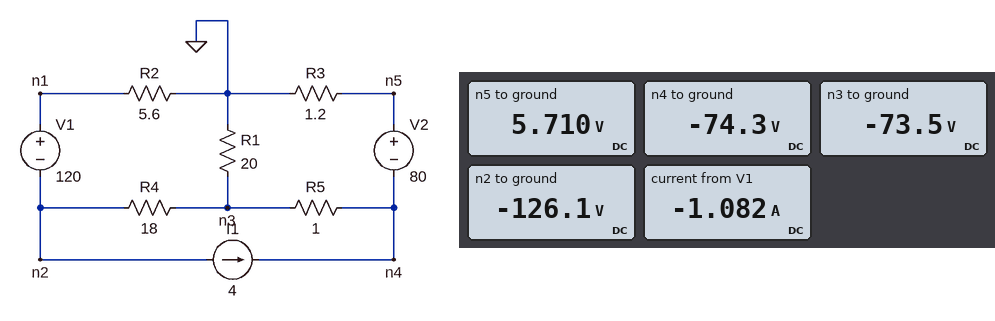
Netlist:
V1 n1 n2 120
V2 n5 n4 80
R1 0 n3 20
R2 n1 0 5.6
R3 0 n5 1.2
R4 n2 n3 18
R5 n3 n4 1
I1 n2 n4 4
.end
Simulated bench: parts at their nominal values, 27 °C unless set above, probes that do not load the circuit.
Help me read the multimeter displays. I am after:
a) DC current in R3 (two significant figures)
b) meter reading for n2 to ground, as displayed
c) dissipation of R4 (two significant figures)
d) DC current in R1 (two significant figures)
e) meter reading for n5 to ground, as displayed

4.8 A
-126.1 V
150 W
3.7 A
5.710 V
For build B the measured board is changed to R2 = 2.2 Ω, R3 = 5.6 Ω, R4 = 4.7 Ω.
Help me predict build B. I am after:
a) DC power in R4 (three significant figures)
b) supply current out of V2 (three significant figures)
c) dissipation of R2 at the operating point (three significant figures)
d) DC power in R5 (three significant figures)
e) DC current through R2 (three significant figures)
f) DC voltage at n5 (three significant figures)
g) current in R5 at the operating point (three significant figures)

244 W
747 mA
22.6 W
10.6 W
3.21 A
4.18 V
3.25 A
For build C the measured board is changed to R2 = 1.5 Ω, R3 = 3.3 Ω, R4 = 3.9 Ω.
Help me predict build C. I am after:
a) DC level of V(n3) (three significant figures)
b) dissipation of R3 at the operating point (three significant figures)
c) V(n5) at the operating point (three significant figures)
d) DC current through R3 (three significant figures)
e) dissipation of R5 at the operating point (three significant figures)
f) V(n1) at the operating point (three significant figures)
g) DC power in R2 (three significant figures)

-83.1 V
145 mW
693 mV
210 mA
14.4 W
5.92 V
23.3 W
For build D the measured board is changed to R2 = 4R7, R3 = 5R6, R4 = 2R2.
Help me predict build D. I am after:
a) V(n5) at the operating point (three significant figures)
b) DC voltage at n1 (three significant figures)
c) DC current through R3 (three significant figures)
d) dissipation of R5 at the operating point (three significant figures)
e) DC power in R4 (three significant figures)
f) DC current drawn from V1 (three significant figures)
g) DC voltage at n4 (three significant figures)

632 mV
19.0 V
113 mA
15.1 W
143 W
4.05 A
-79.4 V
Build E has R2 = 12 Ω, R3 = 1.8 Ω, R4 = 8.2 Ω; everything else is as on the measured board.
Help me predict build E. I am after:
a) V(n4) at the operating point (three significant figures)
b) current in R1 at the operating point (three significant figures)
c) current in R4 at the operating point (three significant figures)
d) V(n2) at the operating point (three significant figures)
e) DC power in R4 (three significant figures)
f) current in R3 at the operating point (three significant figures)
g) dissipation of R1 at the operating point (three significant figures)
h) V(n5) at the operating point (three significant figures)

-74.3 V
3.76 A
4.60 A
-113 V
173 W
3.16 A
282 W
5.69 V
